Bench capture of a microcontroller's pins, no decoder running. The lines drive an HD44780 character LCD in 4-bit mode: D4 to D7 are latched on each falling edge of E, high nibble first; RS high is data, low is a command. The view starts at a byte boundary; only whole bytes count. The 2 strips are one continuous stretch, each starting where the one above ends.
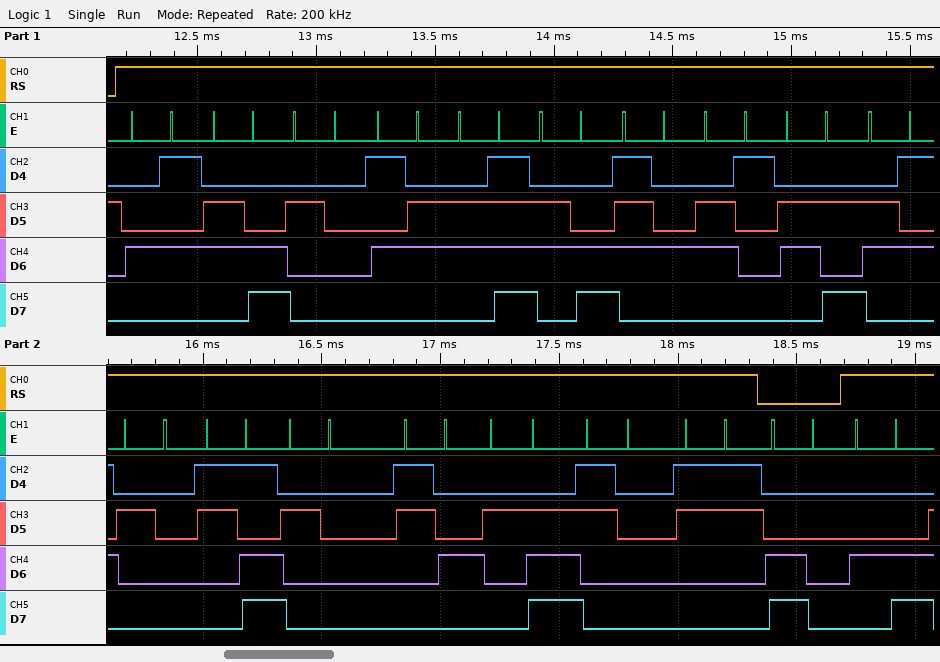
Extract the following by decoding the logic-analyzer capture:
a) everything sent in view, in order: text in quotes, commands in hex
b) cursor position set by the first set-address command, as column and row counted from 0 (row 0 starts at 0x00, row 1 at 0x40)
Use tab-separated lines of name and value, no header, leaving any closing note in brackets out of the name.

everything sent in view, in order: text in quotes, commands in hex	"El Voltaje = 4.03" 0xC0 "L"
cursor position set by the first set-address command, as column and row counted from 0	column 0, row 1
